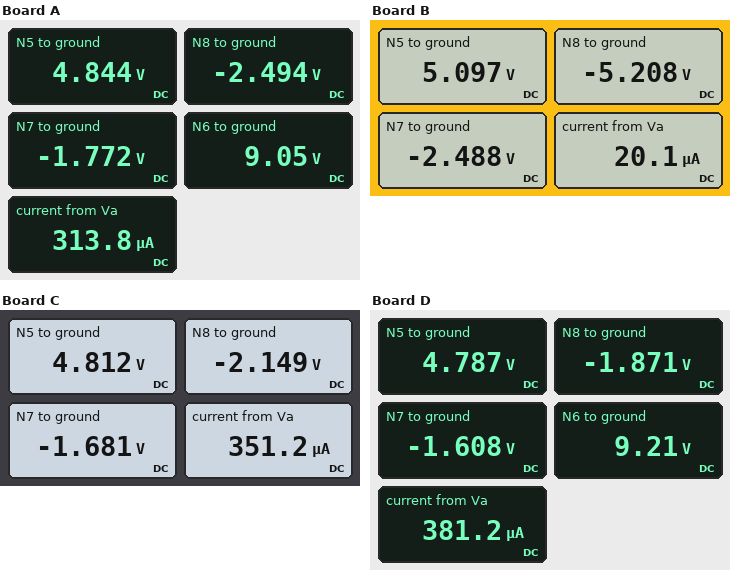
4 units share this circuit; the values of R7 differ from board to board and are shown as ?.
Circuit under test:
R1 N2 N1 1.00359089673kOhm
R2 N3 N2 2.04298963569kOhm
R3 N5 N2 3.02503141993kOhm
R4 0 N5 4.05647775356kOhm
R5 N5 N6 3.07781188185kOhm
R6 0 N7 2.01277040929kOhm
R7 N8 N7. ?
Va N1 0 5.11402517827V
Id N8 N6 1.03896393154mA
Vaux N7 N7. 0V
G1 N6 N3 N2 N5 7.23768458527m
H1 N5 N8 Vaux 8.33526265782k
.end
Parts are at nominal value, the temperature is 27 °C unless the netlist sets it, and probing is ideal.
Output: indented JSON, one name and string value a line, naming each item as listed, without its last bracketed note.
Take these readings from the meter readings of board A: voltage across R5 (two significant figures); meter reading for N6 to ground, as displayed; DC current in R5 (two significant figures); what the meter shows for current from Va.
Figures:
{
  "voltage across R5": "4.2 V",
  "meter reading for N6 to ground, as displayed": "9.05 V",
  "DC current in R5": "1.4 mA",
  "what the meter shows for current from Va": "313.8 µA"
}
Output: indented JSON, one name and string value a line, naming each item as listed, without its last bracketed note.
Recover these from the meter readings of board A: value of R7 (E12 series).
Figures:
{
  "value of R7": "820 Ω"
}
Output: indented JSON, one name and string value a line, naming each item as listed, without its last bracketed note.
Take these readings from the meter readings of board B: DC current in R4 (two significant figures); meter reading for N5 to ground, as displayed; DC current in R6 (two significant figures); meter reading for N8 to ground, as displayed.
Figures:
{
  "DC current in R4": "1.3 mA",
  "meter reading for N5 to ground, as displayed": "5.097 V",
  "DC current in R6": "1.2 mA",
  "meter reading for N8 to ground, as displayed": "-5.208 V"
}
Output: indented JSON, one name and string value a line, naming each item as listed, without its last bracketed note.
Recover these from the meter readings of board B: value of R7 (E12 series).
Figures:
{
  "value of R7": "2.2 kΩ"
}
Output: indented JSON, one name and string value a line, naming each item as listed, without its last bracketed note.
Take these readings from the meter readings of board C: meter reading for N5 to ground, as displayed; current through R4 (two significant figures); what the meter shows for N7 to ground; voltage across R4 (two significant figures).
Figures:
{
  "meter reading for N5 to ground, as displayed": "4.812 V",
  "current through R4": "1.2 mA",
  "what the meter shows for N7 to ground": "-1.681 V",
  "voltage across R4": "4.8 V"
}
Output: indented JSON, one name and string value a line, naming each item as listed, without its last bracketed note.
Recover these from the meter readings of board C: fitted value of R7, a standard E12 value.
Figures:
{
  "fitted value of R7, a standard E12 value": "560 Ω"
}
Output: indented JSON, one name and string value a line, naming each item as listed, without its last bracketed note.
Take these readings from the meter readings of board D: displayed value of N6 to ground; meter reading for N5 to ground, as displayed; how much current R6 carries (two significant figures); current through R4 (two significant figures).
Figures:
{
  "displayed value of N6 to ground": "9.21 V",
  "meter reading for N5 to ground, as displayed": "4.787 V",
  "how much current R6 carries": "800 µA",
  "current through R4": "1.2 mA"
}
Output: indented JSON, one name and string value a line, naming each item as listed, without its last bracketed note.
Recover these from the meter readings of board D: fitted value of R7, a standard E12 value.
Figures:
{
  "fitted value of R7, a standard E12 value": "330 Ω"
}
